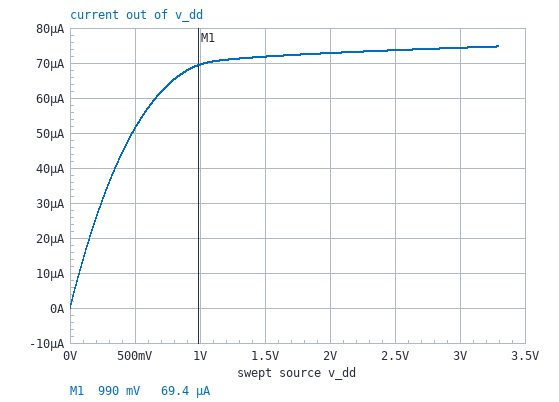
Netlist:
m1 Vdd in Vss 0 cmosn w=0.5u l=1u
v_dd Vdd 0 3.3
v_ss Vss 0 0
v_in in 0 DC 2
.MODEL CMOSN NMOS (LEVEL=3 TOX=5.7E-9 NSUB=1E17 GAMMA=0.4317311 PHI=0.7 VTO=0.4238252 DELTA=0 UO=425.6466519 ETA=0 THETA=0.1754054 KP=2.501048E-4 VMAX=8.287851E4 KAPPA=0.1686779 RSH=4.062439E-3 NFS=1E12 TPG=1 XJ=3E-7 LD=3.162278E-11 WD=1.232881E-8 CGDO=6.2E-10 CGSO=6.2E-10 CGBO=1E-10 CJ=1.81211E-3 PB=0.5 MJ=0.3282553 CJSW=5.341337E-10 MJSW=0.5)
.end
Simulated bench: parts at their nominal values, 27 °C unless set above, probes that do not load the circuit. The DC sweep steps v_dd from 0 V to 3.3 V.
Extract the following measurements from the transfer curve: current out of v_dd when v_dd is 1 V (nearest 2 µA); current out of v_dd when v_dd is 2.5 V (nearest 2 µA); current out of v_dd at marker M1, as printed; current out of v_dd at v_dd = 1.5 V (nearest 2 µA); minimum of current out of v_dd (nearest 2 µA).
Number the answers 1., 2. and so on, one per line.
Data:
1. 70 µA
2. 74 µA
3. 69.4 µA
4. 72 µA
5. 0 A
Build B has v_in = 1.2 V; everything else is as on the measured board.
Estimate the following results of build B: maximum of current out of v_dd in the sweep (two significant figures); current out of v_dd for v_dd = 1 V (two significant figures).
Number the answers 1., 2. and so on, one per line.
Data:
1. 25 µA
2. 24 µA
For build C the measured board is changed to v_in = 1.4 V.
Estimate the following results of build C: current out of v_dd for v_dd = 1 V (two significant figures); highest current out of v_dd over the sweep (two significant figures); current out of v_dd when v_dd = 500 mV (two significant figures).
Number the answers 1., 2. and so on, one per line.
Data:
1. 34 µA
2. 36 µA
3. 30 µA
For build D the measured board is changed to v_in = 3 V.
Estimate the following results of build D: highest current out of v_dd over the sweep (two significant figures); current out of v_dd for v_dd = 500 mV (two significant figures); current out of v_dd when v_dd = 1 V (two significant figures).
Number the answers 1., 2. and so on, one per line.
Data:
1. 150 µA
2. 81 µA
3. 120 µA
